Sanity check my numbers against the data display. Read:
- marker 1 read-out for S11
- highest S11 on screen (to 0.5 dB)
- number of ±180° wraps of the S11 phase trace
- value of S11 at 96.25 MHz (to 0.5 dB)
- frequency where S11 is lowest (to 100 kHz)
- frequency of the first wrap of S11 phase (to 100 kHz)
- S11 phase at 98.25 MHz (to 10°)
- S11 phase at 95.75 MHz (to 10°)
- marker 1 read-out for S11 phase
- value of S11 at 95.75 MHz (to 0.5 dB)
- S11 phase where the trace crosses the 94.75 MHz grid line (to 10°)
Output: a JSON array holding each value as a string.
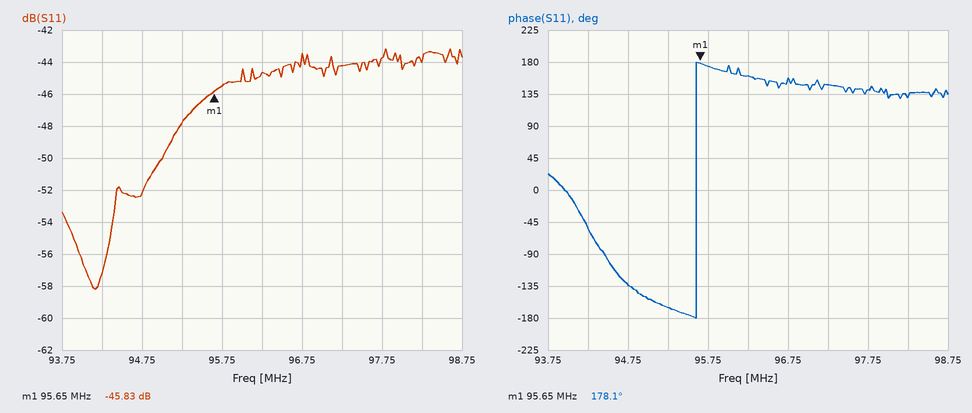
["-45.83 dB", "-43.0 dB", "1", "-44.5 dB", "94.2 MHz", "95.6 MHz", "130°", "170°", "178.1°", "-45.5 dB", "-130°"]
